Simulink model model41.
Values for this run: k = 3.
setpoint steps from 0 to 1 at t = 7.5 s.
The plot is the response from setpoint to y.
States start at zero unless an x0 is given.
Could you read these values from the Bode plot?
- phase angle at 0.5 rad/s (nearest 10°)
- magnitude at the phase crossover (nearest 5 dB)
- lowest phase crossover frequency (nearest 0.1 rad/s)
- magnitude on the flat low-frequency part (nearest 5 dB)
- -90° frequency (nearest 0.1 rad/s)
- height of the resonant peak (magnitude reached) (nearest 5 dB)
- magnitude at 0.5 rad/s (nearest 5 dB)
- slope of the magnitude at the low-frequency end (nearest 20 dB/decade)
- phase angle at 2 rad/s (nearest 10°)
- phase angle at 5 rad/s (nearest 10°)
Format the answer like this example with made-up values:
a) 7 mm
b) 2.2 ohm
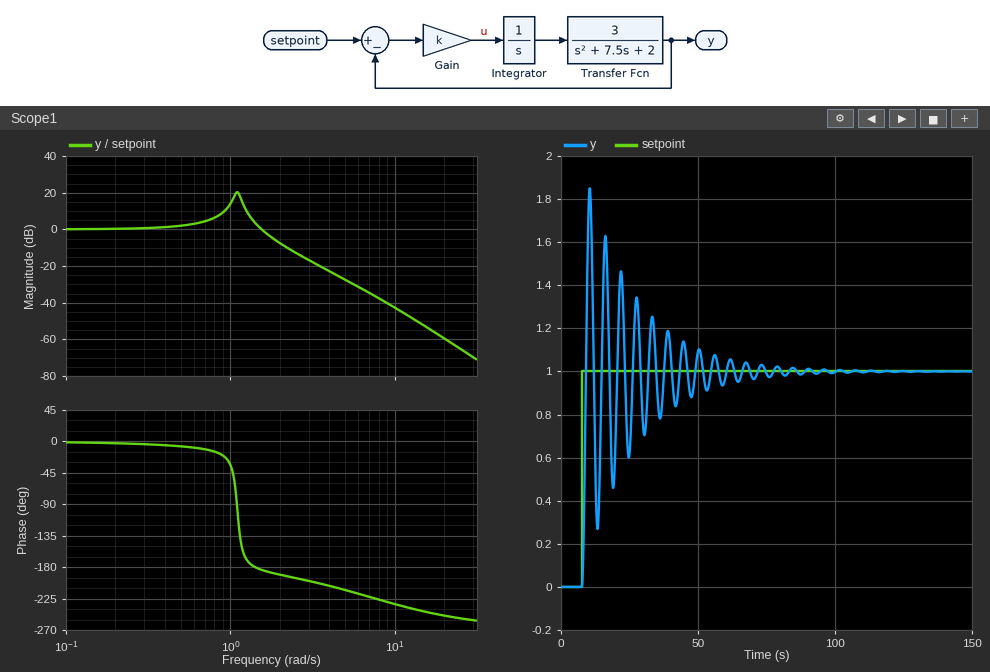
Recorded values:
a) -10°
b) 5 dB
c) 1.4 rad/s
d) 0 dB
e) 1.1 rad/s
f) 20 dB
g) 0 dB
h) 0 dB/decade
i) -190°
j) -210°
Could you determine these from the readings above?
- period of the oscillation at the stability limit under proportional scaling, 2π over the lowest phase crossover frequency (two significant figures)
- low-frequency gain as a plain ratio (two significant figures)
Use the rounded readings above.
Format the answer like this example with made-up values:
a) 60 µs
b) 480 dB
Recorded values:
a) 4.5 s
b) 1.0
